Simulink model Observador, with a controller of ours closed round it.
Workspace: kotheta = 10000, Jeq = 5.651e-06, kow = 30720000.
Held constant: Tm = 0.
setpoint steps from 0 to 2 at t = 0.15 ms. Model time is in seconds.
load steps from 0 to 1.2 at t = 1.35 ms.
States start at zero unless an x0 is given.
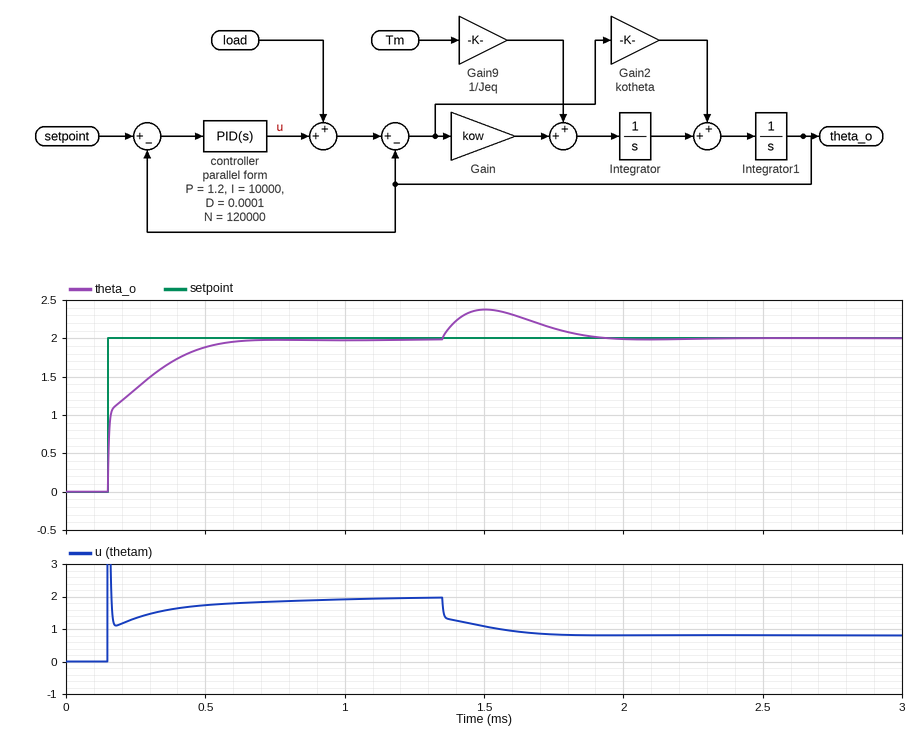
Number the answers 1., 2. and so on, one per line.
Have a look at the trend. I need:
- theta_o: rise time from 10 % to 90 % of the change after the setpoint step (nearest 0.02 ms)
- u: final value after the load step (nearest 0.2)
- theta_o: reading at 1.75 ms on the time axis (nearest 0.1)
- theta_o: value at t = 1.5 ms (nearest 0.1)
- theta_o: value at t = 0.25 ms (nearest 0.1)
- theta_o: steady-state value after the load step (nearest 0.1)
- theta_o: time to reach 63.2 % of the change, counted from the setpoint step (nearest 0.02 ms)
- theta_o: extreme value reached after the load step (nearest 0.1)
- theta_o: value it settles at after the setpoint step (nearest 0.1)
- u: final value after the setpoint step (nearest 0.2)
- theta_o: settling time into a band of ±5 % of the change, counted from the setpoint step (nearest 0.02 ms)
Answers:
1. 0.28 ms
2. 0.8
3. 2.1
4. 2.4
5. 1.3
6. 2.0
7. 0.08 ms
8. 2.4
9. 2.0
10. 2.0
11. 0.36 ms
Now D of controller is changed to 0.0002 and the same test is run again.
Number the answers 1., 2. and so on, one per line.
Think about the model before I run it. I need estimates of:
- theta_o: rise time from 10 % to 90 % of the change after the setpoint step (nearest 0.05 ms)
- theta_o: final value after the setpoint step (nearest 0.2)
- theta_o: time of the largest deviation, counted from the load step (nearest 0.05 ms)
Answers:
1. 0.35 ms
2. 2.0
3. 0.20 ms
